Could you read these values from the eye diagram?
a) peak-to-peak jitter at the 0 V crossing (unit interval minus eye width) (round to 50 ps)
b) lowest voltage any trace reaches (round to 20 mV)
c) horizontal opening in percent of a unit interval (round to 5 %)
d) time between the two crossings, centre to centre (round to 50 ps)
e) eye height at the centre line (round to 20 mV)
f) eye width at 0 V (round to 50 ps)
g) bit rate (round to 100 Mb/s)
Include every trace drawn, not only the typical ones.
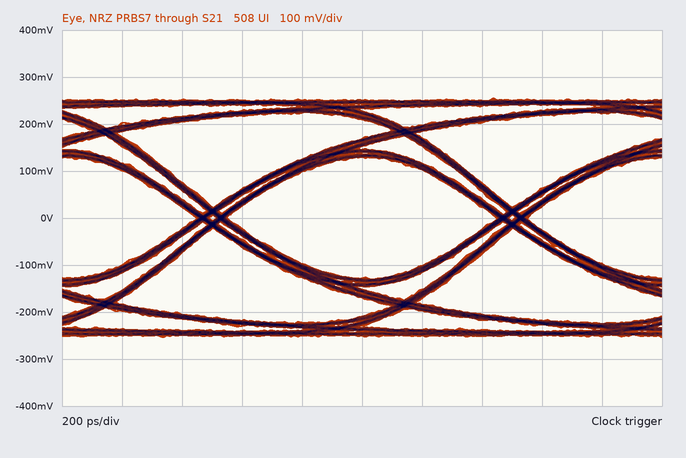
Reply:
100 ps
-260 mV
90 %
1.00 ns
260 mV
900 ps
1.0 Gb/s
